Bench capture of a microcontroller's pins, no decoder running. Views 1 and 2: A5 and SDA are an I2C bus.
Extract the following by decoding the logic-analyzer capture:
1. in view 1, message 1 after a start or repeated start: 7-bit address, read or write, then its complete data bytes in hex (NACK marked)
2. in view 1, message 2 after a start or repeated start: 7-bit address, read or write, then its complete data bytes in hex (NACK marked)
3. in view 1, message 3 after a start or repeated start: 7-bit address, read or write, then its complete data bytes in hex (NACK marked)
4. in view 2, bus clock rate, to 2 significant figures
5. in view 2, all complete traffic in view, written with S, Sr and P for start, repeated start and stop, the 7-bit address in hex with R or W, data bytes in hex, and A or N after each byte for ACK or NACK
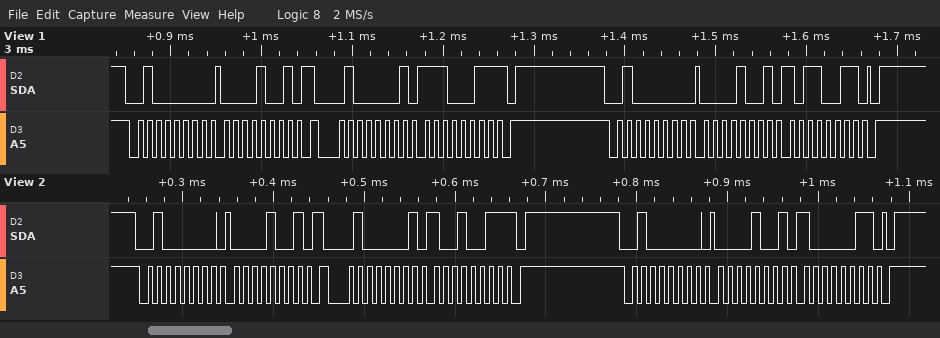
0x20 write: 09
0x20 read: E3 NACK
0x20 write: 09 B3
100 kHz
S 20W A 09 A Sr 20R A 93 N P S 20W A 09 A 83 A P
